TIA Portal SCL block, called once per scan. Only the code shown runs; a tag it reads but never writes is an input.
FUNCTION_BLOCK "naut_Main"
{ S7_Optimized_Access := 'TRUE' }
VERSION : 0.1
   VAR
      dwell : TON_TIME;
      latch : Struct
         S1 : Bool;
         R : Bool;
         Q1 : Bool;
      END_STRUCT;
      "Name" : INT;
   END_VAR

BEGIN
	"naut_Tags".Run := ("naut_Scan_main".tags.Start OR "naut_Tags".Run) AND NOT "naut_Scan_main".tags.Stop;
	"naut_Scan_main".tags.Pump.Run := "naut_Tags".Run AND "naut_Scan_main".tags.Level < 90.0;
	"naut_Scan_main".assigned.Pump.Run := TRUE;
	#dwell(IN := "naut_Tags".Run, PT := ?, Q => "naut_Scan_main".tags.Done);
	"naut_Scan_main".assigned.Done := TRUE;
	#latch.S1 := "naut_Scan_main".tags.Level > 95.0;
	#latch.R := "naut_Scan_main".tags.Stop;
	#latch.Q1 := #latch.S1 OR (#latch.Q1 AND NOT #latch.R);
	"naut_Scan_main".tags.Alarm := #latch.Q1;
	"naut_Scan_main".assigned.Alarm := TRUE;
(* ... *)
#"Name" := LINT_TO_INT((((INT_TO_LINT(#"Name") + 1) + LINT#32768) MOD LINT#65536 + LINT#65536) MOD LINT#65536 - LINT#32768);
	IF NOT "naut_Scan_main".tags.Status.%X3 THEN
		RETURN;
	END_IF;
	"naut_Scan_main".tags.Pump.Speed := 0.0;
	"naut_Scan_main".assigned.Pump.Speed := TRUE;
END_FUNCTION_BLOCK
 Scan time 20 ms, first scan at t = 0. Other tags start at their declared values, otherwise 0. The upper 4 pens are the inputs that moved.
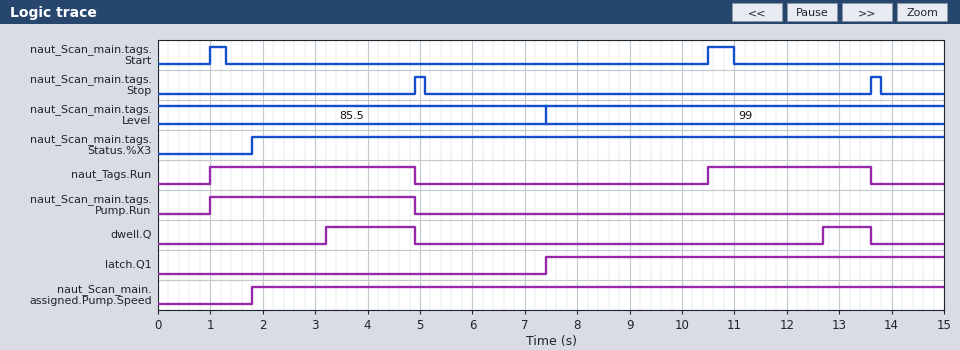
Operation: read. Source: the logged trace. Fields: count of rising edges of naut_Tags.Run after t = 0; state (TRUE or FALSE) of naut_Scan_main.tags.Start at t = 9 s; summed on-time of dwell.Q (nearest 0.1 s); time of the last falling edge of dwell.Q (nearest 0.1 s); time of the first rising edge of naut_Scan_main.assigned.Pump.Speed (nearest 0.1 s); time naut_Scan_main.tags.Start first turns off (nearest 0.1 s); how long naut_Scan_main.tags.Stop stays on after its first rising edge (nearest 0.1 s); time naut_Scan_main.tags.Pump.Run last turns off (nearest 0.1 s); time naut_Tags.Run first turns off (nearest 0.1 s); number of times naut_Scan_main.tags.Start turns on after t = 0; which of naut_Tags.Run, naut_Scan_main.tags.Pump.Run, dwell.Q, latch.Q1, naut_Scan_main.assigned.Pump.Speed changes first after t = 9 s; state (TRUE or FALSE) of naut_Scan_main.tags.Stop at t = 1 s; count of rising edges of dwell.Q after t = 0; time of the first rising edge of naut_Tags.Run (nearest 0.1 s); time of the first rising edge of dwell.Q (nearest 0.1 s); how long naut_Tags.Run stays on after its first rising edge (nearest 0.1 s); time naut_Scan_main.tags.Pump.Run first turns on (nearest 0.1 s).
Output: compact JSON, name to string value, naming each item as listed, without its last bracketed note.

{"count of rising edges of naut_Tags.Run after t = 0": "2", "state (TRUE or FALSE) of naut_Scan_main.tags.Start at t = 9 s": "FALSE", "summed on-time of dwell.Q": "2.6 s", "time of the last falling edge of dwell.Q": "13.6 s", "time of the first rising edge of naut_Scan_main.assigned.Pump.Speed": "1.8 s", "time naut_Scan_main.tags.Start first turns off": "1.3 s", "how long naut_Scan_main.tags.Stop stays on after its first rising edge": "0.2 s", "time naut_Scan_main.tags.Pump.Run last turns off": "4.9 s", "time naut_Tags.Run first turns off": "4.9 s", "number of times naut_Scan_main.tags.Start turns on after t = 0": "2", "which of naut_Tags.Run, naut_Scan_main.tags.Pump.Run, dwell.Q, latch.Q1, naut_Scan_main.assigned.Pump.Speed changes first after t = 9 s": "naut_Tags.Run", "state (TRUE or FALSE) of naut_Scan_main.tags.Stop at t = 1 s": "FALSE", "count of rising edges of dwell.Q after t = 0": "2", "time of the first rising edge of naut_Tags.Run": "1.0 s", "time of the first rising edge of dwell.Q": "3.2 s", "how long naut_Tags.Run stays on after its first rising edge": "3.9 s", "time naut_Scan_main.tags.Pump.Run first turns on": "1.0 s"}
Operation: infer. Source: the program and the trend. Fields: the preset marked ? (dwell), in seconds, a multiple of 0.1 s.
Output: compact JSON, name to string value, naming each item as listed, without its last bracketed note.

{"the preset marked ? (dwell), in seconds, a multiple of 0.1 s": "2.2 s"}
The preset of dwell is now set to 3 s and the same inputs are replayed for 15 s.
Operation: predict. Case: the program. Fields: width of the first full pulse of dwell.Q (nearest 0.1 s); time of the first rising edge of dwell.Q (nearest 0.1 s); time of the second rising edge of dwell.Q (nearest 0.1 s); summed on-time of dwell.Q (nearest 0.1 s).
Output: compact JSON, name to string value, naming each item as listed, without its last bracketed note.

{"width of the first full pulse of dwell.Q": "0.9 s", "time of the first rising edge of dwell.Q": "4.0 s", "time of the second rising edge of dwell.Q": "13.5 s", "summed on-time of dwell.Q": "1.0 s"}
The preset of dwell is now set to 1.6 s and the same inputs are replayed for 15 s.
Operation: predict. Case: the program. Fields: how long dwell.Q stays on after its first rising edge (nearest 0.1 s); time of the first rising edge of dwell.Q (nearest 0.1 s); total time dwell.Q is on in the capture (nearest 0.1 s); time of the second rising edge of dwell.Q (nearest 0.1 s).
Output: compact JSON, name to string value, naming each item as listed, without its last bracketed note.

{"how long dwell.Q stays on after its first rising edge": "2.3 s", "time of the first rising edge of dwell.Q": "2.6 s", "total time dwell.Q is on in the capture": "3.8 s", "time of the second rising edge of dwell.Q": "12.1 s"}
